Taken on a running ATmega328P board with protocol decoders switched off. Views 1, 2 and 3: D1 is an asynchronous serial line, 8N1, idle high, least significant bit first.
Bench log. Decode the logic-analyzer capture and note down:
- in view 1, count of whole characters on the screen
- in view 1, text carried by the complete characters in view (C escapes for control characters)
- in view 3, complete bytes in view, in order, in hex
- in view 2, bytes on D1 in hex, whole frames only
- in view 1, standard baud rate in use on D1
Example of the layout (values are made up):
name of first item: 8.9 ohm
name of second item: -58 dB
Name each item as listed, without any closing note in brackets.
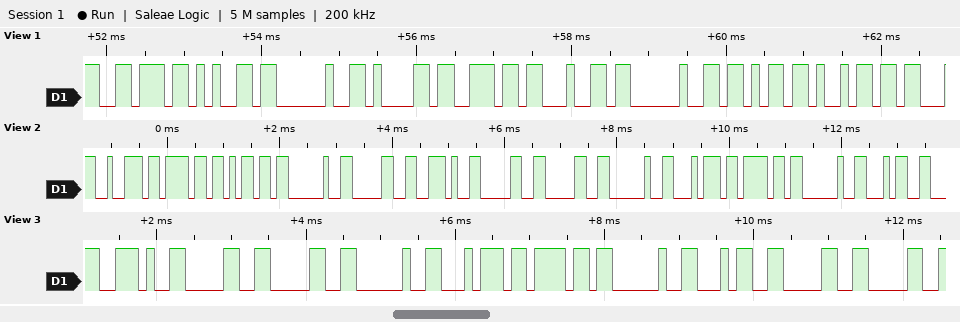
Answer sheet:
in view 1, count of whole characters on the screen: 9
in view 1, text carried by the complete characters in view: "ve and ki"
in view 3, complete bytes in view, in order, in hex: 2E 30 30 20 74 6F 20 34 30 30
in view 2, bytes on D1 in hex, whole frames only: 0x72 0x6F 0x6D 0x20 0x30 0x2E 0x30 0x30 0x20 0x74 0x6F 0x20 0x34
in view 1, standard baud rate in use on D1: 9600 baud
